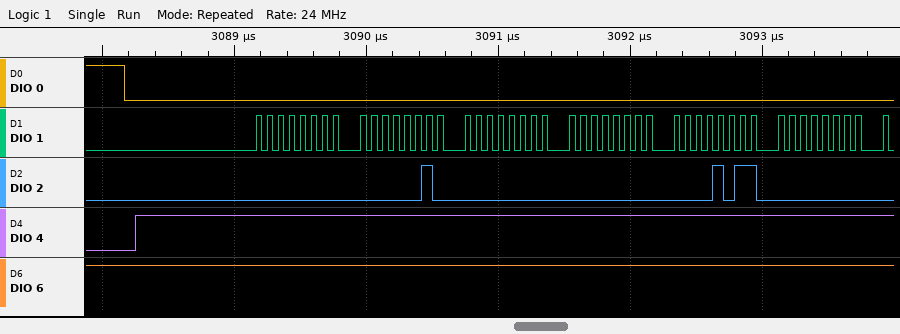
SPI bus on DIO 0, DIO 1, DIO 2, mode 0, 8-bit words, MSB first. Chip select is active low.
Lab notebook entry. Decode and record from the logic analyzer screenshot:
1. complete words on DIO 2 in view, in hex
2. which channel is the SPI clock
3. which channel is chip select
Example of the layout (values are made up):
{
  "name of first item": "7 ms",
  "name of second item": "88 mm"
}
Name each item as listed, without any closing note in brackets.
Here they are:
{
  "complete words on DIO 2 in view, in hex": "00, 02, 00, 00, 0B, 00",
  "which channel is the SPI clock": "DIO 1",
  "which channel is chip select": "DIO 0"
}
